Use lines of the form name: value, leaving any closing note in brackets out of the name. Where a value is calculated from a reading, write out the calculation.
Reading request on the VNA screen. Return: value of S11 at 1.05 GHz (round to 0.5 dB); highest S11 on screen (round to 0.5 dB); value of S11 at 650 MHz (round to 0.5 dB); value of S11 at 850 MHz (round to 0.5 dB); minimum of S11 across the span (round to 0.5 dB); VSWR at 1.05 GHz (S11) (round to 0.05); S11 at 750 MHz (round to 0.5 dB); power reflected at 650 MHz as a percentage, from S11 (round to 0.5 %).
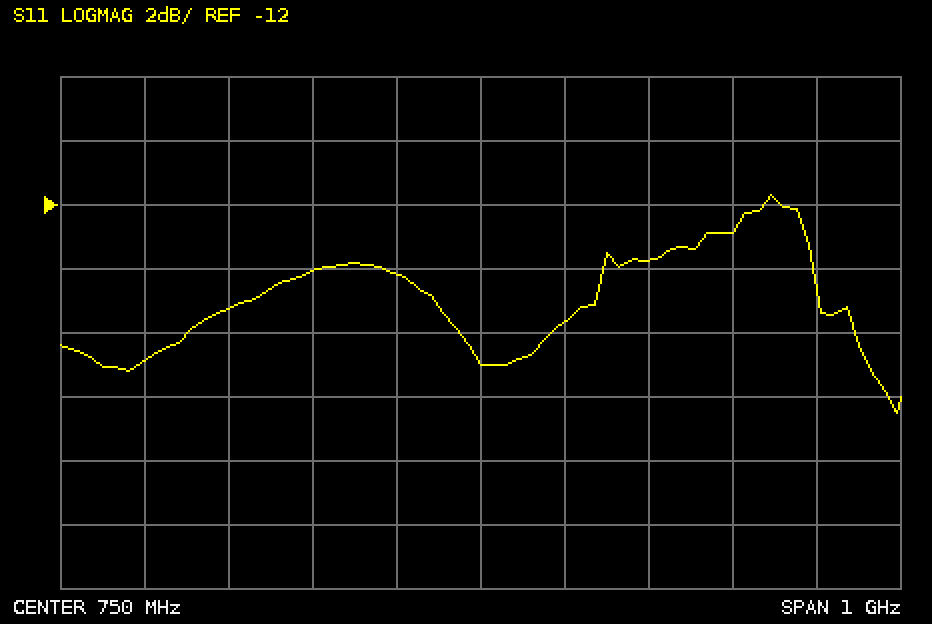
value of S11 at 1.05 GHz: -13.0 dB
highest S11 on screen: -11.5 dB
value of S11 at 650 MHz: -14.0 dB
value of S11 at 850 MHz: -15.5 dB
minimum of S11 across the span: -18.5 dB
VSWR at 1.05 GHz (S11): |Γ| = 10^(-13/20) = 0.2239; VSWR = (1 + 0.2239)/(1 − 0.2239) ≈ 1.58, so 1.60 to the nearest 0.05
S11 at 750 MHz: -17.0 dB
power reflected at 650 MHz as a percentage, from S11: 10^(-14/10) ≈ 4.0 %
